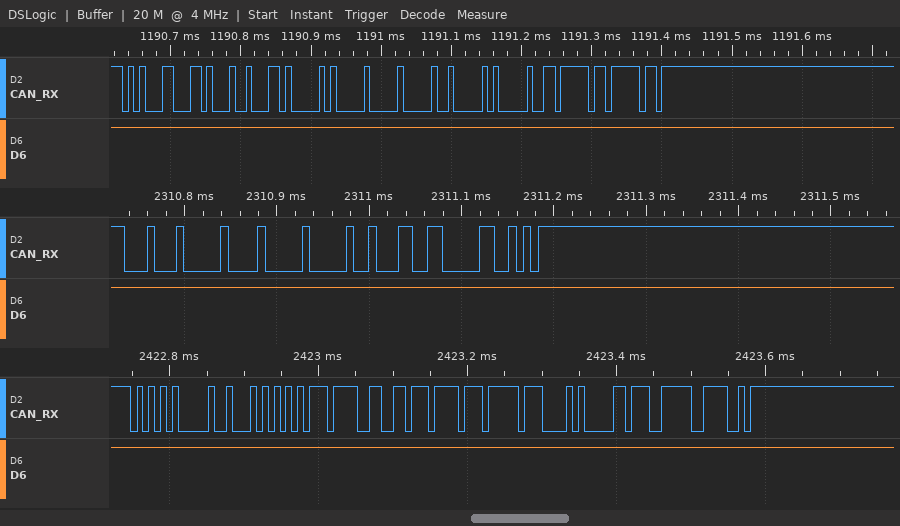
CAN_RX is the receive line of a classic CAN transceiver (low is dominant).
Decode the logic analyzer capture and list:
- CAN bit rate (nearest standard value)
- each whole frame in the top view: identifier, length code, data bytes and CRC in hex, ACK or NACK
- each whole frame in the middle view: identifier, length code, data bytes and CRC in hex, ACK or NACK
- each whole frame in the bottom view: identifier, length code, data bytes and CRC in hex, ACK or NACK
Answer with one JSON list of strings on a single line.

["125 kbit/s", "ID 14611234, DLC 4, data 00 01 02 03, CRC 3FBF, ACK", "ID 110, DLC 2, data 00 11, CRC 4C12, ACK", "ID 550, DLC 8, data AA BB CC DD EE FF 0A 0B, CRC 4FBC, ACK"]
